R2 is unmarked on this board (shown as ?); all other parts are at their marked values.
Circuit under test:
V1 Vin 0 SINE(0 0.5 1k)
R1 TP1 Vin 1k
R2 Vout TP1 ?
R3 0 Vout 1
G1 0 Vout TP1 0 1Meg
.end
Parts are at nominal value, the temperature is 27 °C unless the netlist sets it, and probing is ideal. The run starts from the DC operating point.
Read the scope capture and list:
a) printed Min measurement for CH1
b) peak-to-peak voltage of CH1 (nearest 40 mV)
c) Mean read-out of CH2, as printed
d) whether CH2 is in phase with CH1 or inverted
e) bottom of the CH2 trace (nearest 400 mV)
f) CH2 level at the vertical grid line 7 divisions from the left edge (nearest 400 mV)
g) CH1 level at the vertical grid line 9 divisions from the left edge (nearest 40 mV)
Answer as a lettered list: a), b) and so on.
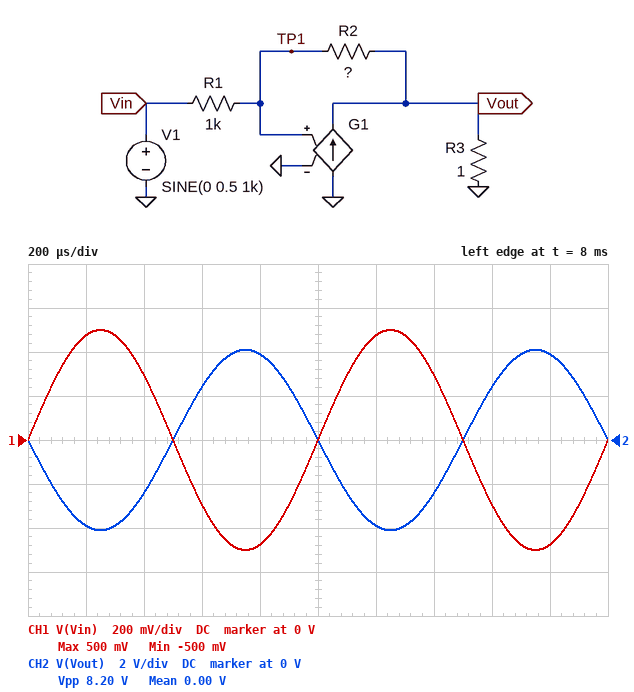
a) -500 mV
b) 1.00 V
c) 0.00 V
d) inverted
e) -4.0 V
f) -2.4 V
g) -480 mV
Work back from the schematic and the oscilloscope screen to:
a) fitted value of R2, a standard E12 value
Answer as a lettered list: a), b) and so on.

a) 8.2 kΩ
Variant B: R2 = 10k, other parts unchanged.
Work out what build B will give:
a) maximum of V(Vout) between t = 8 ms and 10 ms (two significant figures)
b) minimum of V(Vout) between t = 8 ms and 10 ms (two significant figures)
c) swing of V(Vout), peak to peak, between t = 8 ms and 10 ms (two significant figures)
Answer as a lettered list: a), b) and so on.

a) 5.0 V
b) -5.0 V
c) 10 V
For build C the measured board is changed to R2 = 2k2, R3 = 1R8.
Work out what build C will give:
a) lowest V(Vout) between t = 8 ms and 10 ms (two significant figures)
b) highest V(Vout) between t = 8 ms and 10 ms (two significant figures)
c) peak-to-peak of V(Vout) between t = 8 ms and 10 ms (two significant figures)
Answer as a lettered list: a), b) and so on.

a) -1.1 V
b) 1.1 V
c) 2.2 V
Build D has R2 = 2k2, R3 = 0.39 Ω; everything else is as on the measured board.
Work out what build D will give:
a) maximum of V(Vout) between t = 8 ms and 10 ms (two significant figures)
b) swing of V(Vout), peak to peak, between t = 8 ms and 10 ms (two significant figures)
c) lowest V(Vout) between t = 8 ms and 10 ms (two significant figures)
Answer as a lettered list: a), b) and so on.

a) 1.1 V
b) 2.2 V
c) -1.1 V
